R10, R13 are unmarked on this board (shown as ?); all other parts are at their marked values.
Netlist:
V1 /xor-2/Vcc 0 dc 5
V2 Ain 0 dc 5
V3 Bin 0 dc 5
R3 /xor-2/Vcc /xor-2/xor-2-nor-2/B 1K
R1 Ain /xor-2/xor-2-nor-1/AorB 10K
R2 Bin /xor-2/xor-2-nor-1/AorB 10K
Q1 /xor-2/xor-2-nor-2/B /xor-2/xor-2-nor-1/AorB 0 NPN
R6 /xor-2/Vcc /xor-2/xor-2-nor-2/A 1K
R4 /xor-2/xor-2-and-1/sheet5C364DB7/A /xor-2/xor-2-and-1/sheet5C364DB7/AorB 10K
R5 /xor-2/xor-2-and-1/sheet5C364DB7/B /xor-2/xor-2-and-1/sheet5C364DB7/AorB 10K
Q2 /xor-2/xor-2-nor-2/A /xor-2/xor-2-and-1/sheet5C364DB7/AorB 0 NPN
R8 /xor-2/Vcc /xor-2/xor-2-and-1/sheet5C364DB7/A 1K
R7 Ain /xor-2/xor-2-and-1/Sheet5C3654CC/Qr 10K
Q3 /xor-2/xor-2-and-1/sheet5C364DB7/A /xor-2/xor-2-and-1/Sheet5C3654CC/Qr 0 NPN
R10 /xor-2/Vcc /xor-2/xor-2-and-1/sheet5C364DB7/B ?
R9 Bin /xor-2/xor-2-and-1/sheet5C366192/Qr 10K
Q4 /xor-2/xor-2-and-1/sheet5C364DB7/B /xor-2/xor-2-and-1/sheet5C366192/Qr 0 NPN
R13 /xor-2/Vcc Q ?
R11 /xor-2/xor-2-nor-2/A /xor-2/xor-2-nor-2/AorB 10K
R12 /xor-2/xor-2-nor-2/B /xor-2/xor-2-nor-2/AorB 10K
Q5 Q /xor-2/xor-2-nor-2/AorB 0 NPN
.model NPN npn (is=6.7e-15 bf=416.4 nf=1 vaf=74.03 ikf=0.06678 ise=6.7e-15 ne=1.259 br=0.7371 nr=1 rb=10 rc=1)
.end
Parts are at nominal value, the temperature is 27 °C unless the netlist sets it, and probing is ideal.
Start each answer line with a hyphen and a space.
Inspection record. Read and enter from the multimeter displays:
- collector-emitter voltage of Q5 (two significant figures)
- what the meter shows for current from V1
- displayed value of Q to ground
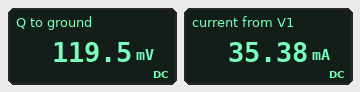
- 120 mV
- 35.38 mA
- 119.5 mV
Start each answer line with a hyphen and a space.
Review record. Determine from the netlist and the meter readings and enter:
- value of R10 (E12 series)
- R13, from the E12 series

- 330 Ω
- 470 Ω
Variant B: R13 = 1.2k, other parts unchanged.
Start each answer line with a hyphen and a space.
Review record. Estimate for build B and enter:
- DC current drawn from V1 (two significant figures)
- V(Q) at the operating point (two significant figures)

- 29 mA
- 85 mV
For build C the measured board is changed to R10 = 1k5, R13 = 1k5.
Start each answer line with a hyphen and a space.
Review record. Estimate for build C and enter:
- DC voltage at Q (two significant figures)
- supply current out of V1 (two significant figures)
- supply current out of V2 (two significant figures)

- 78 mV
- 17 mA
- 860 µA
